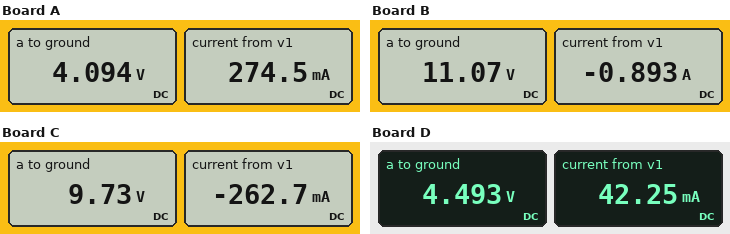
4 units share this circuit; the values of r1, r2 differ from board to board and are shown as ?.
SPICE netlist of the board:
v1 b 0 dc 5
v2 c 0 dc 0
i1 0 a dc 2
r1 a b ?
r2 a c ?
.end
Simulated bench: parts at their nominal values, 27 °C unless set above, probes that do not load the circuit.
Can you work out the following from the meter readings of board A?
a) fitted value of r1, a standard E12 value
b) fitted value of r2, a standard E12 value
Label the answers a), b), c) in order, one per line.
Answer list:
a) 3.3 Ω
b) 1.8 Ω
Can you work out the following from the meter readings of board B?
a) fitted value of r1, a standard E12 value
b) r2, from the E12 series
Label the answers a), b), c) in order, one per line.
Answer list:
a) 6.8 Ω
b) 10 Ω
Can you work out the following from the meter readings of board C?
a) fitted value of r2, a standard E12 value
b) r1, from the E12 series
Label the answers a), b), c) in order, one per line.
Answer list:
a) 5.6 Ω
b) 18 Ω
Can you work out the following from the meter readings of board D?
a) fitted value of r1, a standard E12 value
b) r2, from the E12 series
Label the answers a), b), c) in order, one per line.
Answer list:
a) 12 Ω
b) 2.2 Ω
